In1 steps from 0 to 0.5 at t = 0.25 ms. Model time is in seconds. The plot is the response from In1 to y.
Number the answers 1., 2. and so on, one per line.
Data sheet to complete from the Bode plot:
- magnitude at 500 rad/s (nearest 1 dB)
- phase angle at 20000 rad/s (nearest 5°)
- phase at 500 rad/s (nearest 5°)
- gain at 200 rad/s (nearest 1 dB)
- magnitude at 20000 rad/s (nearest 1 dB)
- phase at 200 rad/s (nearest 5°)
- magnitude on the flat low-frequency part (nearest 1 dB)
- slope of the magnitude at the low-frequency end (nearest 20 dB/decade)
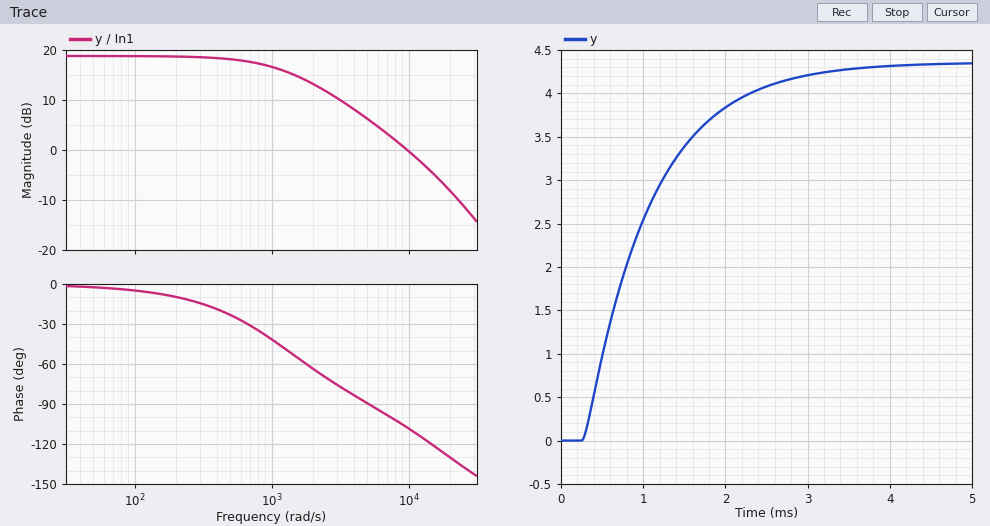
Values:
1. 18 dB
2. -130°
3. -25°
4. 19 dB
5. -8 dB
6. -10°
7. 19 dB
8. 0 dB/decade
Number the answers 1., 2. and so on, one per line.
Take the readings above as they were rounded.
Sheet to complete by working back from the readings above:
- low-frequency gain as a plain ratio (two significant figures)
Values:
1. 8.9
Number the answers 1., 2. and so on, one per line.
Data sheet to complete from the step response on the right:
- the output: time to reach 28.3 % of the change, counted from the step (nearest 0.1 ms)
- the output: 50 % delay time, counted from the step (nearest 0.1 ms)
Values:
1. 0.3 ms
2. 0.6 ms
